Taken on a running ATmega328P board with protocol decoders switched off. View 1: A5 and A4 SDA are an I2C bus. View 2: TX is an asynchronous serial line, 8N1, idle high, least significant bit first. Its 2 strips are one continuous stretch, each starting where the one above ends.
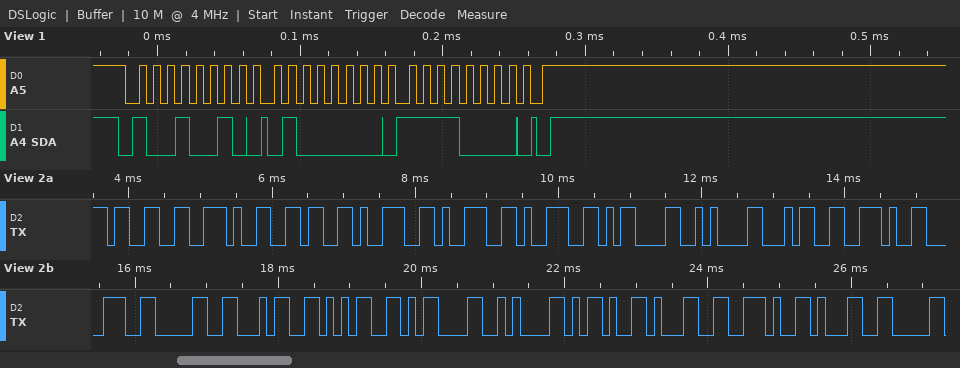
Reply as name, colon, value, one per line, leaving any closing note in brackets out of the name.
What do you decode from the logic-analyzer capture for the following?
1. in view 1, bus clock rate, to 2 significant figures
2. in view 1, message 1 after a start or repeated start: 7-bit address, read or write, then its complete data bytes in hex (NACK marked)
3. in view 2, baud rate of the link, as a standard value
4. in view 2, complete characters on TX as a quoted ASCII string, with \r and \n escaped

in view 1, bus clock rate, to 2 significant figures: 100 kHz
in view 1, message 1 after a start or repeated start: 7-bit address, read or write, then its complete data bytes in hex: 0x49 write: 40 F0
in view 2, baud rate of the link, as a standard value: 9600 baud
in view 2, complete characters on TX as a quoted ASCII string, with \r and \n escaped: "3.6999\r\n4.8045\r\n-1.1"
